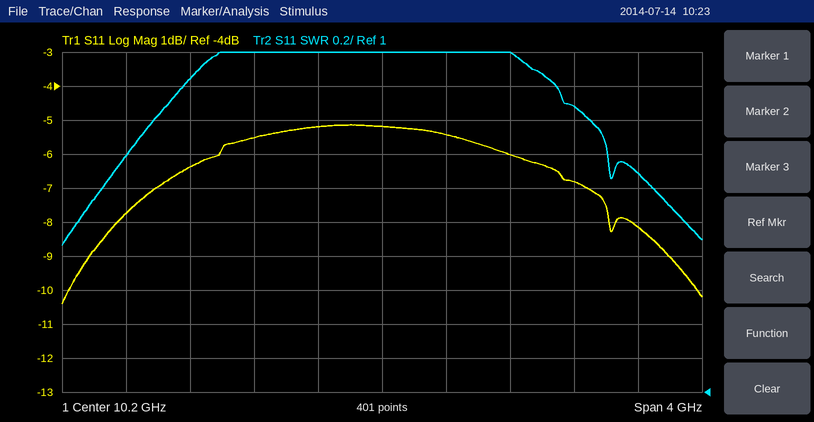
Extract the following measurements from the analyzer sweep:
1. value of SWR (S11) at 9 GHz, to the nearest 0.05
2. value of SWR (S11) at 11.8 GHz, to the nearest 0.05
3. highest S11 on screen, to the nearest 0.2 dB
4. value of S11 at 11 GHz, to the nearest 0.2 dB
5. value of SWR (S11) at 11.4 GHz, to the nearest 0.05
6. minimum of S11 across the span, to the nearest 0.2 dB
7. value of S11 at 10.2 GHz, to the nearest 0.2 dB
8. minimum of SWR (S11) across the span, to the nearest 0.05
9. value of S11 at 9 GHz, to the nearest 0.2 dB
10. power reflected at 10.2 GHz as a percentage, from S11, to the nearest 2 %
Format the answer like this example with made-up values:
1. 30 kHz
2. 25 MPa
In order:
1. 2.85
2. 2.30
3. -5.2 dB
4. -6.0 dB
5. 2.70
6. -10.4 dB
7. -5.2 dB
8. 1.85
9. -6.4 dB
10. 30 %
